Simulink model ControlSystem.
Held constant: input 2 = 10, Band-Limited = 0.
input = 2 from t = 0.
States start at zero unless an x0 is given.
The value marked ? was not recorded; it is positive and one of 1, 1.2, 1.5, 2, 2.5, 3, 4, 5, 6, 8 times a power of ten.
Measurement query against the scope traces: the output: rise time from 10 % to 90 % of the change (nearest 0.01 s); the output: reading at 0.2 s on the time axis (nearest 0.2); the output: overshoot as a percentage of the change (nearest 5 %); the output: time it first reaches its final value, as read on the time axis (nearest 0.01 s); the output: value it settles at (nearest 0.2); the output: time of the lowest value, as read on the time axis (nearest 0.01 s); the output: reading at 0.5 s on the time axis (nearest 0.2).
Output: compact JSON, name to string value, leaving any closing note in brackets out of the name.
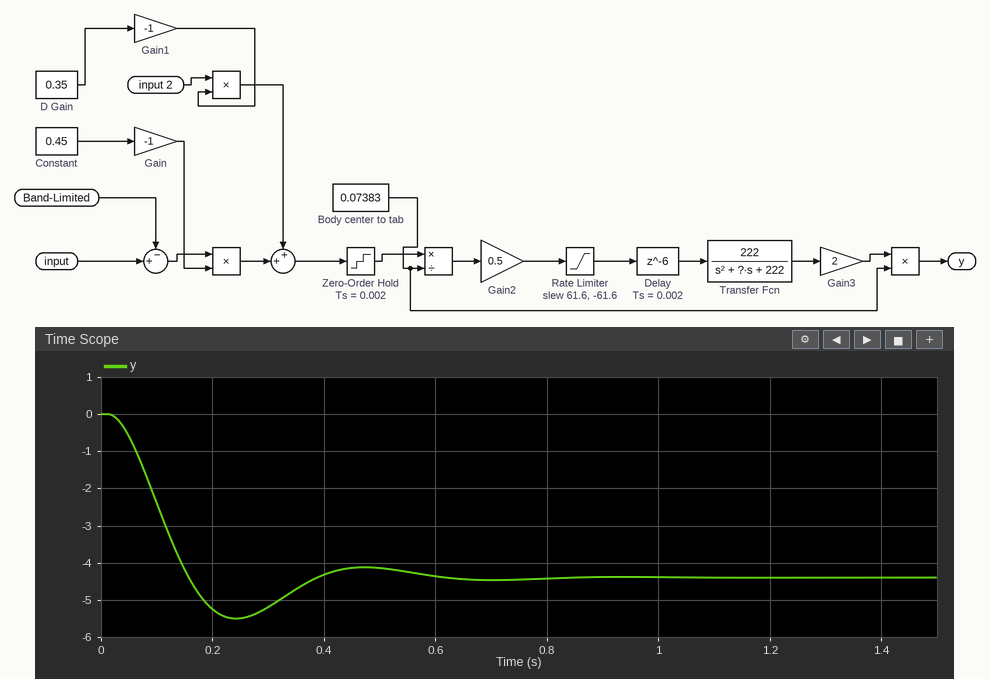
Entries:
{"the output: rise time from 10 % to 90 % of the change": "0.10 s", "the output: reading at 0.2 s on the time axis": "-5.2", "the output: overshoot as a percentage of the change": "25 %", "the output: time it first reaches its final value, as read on the time axis": "0.16 s", "the output: value it settles at": "-4.4", "the output: time of the lowest value, as read on the time axis": "0.24 s", "the output: reading at 0.5 s on the time axis": "-4.2"}
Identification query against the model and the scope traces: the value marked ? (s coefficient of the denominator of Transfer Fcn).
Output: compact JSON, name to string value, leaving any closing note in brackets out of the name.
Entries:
{"the value marked ?": "12"}
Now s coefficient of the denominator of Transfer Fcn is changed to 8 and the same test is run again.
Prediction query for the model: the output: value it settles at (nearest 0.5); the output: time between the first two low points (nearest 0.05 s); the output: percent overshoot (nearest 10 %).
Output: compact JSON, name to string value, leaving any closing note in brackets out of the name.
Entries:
{"the output: value it settles at": "-4.5", "the output: time between the first two low points": "0.45 s", "the output: percent overshoot": "40 %"}
